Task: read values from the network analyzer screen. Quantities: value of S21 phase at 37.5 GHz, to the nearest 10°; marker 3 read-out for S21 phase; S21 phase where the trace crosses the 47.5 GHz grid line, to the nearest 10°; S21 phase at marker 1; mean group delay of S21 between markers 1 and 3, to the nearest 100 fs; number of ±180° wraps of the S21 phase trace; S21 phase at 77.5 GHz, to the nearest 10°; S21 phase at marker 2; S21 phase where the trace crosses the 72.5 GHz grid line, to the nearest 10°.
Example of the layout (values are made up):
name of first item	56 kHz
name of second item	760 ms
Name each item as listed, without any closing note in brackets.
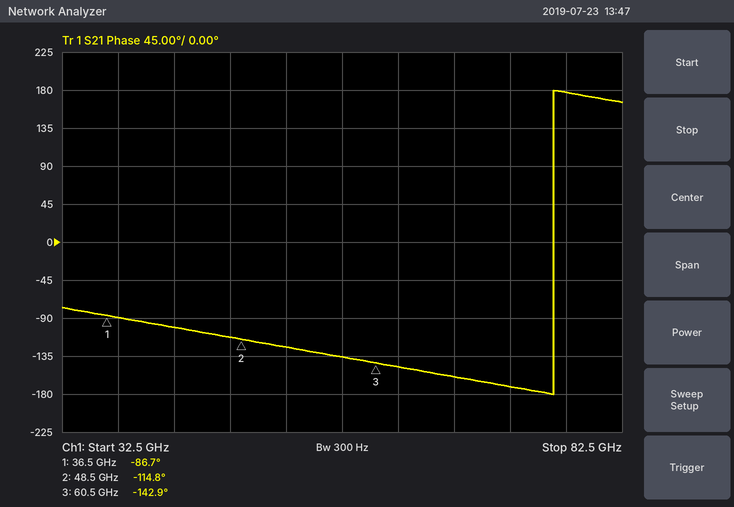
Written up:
value of S21 phase at 37.5 GHz, to the nearest 10°	-90°
marker 3 read-out for S21 phase	-142.9°
S21 phase where the trace crosses the 47.5 GHz grid line, to the nearest 10°	-110°
S21 phase at marker 1	-86.7°
mean group delay of S21 between markers 1 and 3, to the nearest 100 fs	6.5 ps
number of ±180° wraps of the S21 phase trace	1
S21 phase at 77.5 GHz, to the nearest 10°	180°
S21 phase at marker 2	-114.8°
S21 phase where the trace crosses the 72.5 GHz grid line, to the nearest 10°	-170°
